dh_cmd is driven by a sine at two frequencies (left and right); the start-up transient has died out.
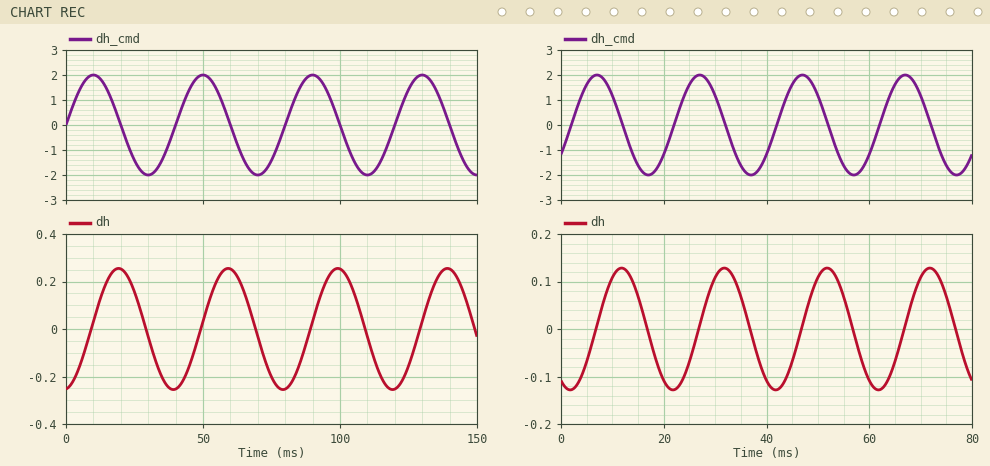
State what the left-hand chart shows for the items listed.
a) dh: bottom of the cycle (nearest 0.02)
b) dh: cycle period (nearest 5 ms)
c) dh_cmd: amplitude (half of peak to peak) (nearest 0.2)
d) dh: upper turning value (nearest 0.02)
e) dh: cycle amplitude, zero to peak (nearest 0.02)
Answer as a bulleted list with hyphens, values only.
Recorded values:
- -0.26
- 40 ms
- 2.0
- 0.26
- 0.26
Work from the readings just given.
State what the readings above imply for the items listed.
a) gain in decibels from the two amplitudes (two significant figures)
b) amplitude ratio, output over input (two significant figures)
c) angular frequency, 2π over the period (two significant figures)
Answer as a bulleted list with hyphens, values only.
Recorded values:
- -18 dB
- 0.13
- 0.16 rad/ms
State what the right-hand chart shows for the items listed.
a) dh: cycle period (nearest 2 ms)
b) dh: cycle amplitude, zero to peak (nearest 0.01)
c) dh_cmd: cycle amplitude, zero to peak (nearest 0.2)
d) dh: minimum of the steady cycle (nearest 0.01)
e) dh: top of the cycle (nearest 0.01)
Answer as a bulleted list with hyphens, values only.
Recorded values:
- 20 ms
- 0.13
- 2.0
- -0.13
- 0.13
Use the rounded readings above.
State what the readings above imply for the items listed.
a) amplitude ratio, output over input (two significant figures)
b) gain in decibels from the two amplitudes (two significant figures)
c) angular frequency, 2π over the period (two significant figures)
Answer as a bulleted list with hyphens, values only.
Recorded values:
- 0.065
- -24 dB
- 0.31 rad/ms
